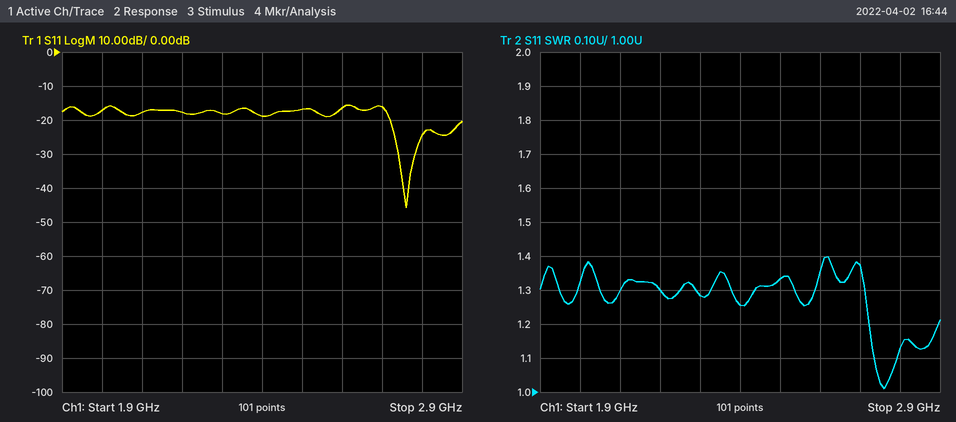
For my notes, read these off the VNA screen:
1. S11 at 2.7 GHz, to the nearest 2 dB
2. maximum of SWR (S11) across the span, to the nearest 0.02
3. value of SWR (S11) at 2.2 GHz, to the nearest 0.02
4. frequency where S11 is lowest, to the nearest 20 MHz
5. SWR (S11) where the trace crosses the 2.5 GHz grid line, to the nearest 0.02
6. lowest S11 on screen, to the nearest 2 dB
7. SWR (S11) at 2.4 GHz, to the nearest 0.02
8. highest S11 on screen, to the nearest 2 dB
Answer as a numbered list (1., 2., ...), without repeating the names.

1. -16 dB
2. 1.40
3. 1.30
4. 2.76 GHz
5. 1.34
6. -46 dB
7. 1.26
8. -16 dB
